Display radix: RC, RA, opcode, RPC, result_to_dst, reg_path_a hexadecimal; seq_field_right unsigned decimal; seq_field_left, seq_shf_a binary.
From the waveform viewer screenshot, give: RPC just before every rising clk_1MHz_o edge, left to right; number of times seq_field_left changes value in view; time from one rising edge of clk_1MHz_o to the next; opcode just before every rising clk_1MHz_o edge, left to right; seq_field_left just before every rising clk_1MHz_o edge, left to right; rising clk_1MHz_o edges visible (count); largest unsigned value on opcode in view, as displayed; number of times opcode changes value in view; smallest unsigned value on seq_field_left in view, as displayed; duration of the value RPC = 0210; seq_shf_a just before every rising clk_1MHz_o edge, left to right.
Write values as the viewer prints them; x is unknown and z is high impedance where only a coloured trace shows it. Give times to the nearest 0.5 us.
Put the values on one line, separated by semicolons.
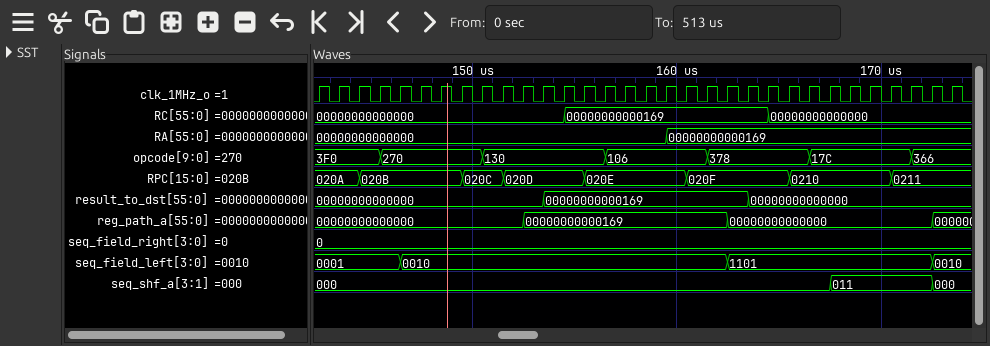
020A, 020A, 020A, 020B, 020B, 020B, 020B, 020B, 020C, 020C, 020D, 020D, 020D, 020D, 020E, 020E, 020E, 020E, 020E, 020F, 020F, 020F, 020F, 020F, 0210, 0210, 0210, 0210, 0210, 0211, 0211, 0211; 3; 1 us; 3F0, 3F0, 3F0, 3F0, 270, 270, 270, 270, 270, 130, 130, 130, 130, 130, 130, 106, 106, 106, 106, 106, 378, 378, 378, 378, 378, 17C, 17C, 17C, 17C, 17C, 366, 366; 0001, 0001, 0001, 0001, 0001, 0010, 0010, 0010, 0010, 0010, 0010, 0010, 0010, 0010, 0010, 0010, 0010, 0010, 0010, 0010, 0010, 1101, 1101, 1101, 1101, 1101, 1101, 1101, 1101, 1101, 1101, 0010; 32; 3F0; 6; 0001; 5 us; 000, 000, 000, 000, 000, 000, 000, 000, 000, 000, 000, 000, 000, 000, 000, 000, 000, 000, 000, 000, 000, 000, 000, 000, 000, 000, 011, 011, 011, 011, 011, 000
